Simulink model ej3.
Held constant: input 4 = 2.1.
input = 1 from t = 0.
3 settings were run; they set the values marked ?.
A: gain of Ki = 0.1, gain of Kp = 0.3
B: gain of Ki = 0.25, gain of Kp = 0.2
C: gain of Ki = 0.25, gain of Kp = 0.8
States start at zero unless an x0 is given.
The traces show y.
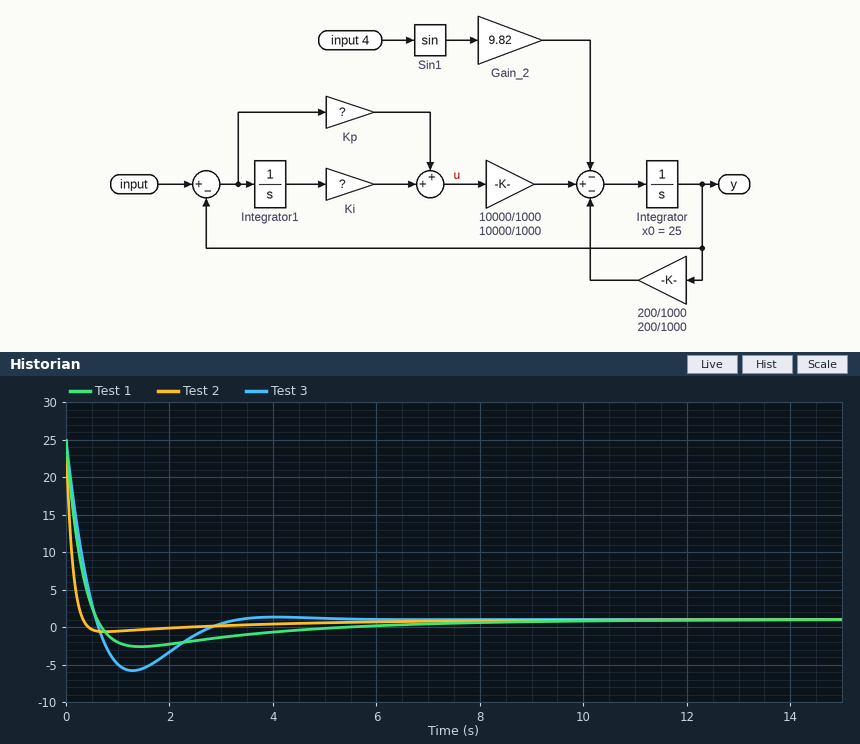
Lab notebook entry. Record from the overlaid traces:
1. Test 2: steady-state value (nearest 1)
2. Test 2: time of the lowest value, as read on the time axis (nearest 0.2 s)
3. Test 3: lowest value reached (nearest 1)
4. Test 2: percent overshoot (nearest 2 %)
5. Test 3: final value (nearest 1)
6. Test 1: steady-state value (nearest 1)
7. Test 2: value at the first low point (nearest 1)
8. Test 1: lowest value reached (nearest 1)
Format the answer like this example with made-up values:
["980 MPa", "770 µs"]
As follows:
["1", "0.8 s", "-6", "6 %", "1", "1", "-1", "-3"]
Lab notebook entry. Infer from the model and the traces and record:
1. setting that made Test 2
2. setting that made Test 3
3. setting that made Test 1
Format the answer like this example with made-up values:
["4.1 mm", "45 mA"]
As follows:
["C", "B", "A"]
